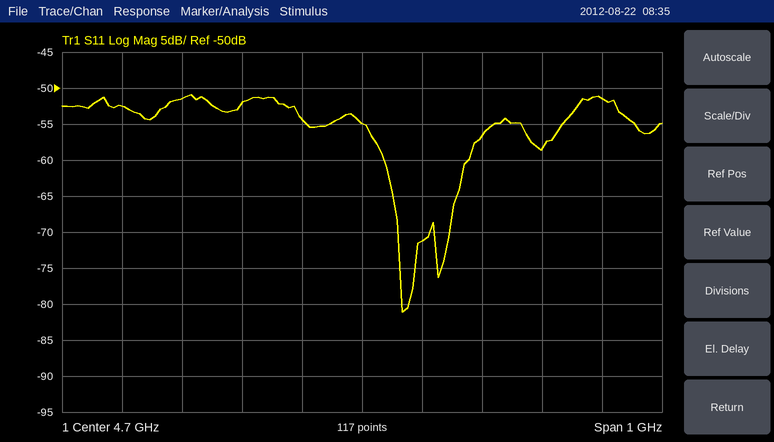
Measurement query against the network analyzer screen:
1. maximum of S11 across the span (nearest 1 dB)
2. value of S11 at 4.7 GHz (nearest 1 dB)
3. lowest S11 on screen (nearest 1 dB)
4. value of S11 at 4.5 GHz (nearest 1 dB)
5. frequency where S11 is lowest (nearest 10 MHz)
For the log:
-51 dB
-55 dB
-81 dB
-52 dB
4.77 GHz
